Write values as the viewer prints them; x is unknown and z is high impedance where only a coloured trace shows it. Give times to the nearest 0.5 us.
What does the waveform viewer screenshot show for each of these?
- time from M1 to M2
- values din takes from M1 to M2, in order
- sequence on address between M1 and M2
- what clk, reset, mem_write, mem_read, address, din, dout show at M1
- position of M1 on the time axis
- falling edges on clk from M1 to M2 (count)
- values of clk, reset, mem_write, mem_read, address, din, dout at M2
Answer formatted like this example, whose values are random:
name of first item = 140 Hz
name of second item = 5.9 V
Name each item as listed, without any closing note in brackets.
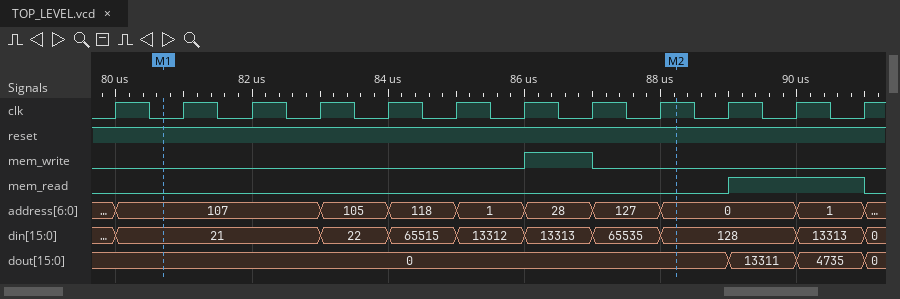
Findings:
time from M1 to M2 = 7.5 us
values din takes from M1 to M2, in order = 21, 22, 65515, 13312, 13313, 65535, 128
sequence on address between M1 and M2 = 107, 105, 118, 1, 28, 127, 0
what clk, reset, mem_write, mem_read, address, din, dout show at M1 = clk=0, reset=1, mem_write=0, mem_read=0, address=107, din=21, dout=0
position of M1 on the time axis = 80.5 us
falling edges on clk from M1 to M2 = 7
values of clk, reset, mem_write, mem_read, address, din, dout at M2 = clk=1, reset=1, mem_write=0, mem_read=0, address=0, din=128, dout=0
